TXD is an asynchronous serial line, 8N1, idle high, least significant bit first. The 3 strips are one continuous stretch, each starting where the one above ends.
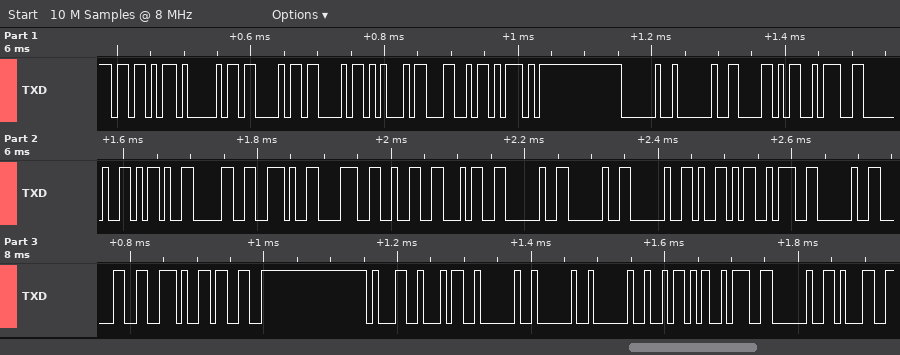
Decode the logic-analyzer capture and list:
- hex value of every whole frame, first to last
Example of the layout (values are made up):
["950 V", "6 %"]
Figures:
["5B 41 43 43 45 4C 5D 20 20 58 3A 20 2D 30 2E 38 32 34 20 20 20 59 3A 20 30 2E 33 31 34 20 20 20 5A 3A 20 31"]
